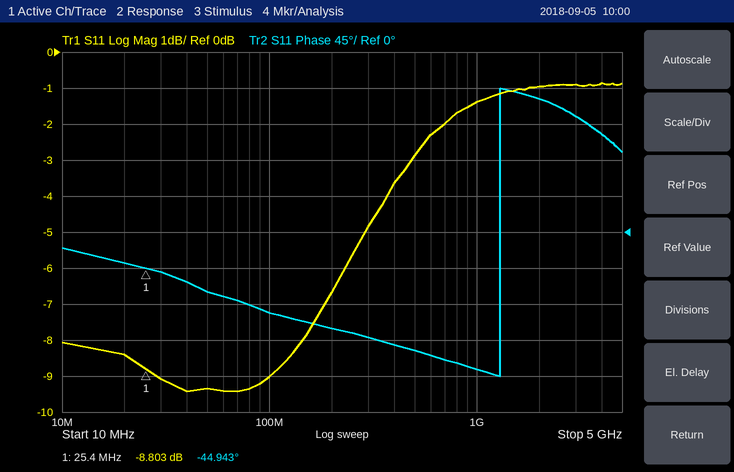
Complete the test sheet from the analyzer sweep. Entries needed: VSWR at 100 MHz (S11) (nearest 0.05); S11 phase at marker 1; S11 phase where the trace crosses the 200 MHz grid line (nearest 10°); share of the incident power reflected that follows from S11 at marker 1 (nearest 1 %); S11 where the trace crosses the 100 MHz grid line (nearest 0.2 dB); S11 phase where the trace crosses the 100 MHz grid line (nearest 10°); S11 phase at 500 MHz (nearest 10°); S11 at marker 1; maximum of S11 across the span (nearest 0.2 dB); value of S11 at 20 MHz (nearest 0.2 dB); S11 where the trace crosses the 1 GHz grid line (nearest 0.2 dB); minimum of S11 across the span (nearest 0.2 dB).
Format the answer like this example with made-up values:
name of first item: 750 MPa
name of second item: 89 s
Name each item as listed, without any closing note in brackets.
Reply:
VSWR at 100 MHz (S11): 2.10
S11 phase at marker 1: -44.943°
S11 phase where the trace crosses the 200 MHz grid line: -120°
share of the incident power reflected that follows from S11 at marker 1: 13 %
S11 where the trace crosses the 100 MHz grid line: -9.0 dB
S11 phase where the trace crosses the 100 MHz grid line: -100°
S11 phase at 500 MHz: -150°
S11 at marker 1: -8.803 dB
maximum of S11 across the span: -0.8 dB
value of S11 at 20 MHz: -8.4 dB
S11 where the trace crosses the 1 GHz grid line: -1.4 dB
minimum of S11 across the span: -9.4 dB
